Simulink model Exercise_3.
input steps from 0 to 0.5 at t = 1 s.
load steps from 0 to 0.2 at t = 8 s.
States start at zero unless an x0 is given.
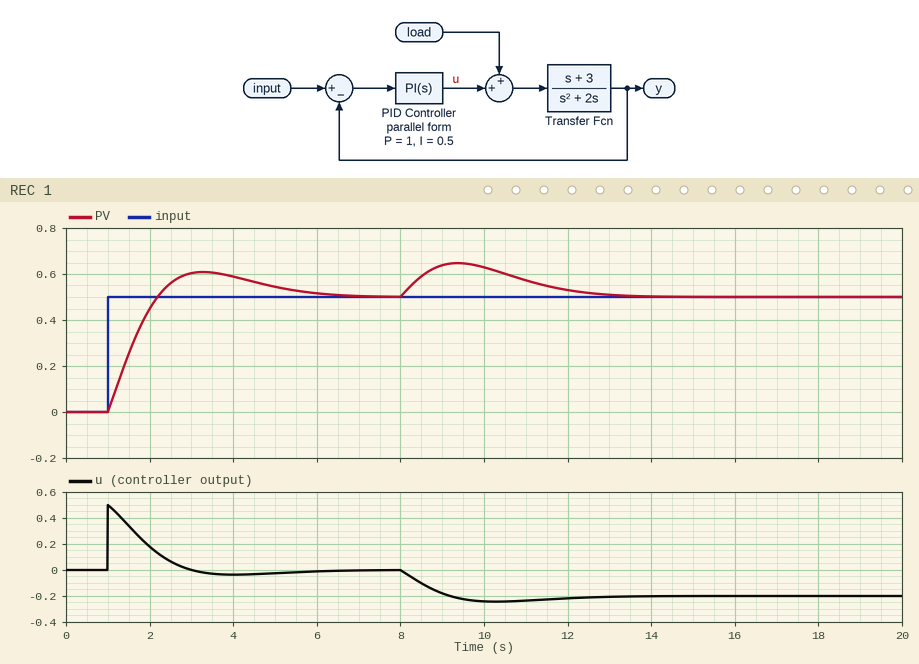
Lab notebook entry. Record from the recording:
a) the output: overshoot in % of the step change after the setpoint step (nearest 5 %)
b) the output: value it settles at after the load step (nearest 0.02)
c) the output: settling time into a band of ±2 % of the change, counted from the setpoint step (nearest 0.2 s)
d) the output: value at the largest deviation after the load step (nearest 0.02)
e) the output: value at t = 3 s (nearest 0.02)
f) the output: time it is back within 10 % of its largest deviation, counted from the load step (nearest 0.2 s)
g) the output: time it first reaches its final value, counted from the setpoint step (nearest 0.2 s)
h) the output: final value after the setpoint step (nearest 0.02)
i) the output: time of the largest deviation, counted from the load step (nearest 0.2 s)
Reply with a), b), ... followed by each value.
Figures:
a) 20 %
b) 0.50
c) 5.4 s
d) 0.64
e) 0.60
f) 4.6 s
g) 1.2 s
h) 0.50
i) 1.4 s
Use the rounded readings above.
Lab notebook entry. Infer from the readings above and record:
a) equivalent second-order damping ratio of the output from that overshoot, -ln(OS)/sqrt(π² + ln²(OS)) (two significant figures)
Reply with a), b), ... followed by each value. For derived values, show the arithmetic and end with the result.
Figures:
a) ln(0.2) = -1.609; 1.609 / sqrt(9.870 + 2.590) = 0.46
